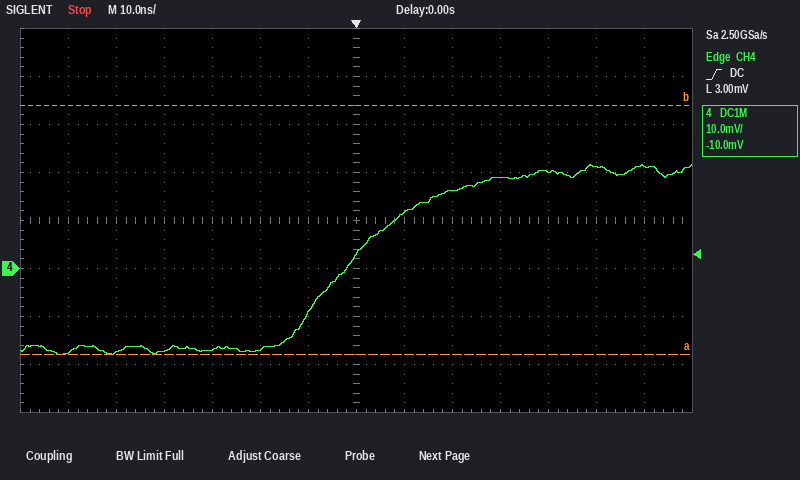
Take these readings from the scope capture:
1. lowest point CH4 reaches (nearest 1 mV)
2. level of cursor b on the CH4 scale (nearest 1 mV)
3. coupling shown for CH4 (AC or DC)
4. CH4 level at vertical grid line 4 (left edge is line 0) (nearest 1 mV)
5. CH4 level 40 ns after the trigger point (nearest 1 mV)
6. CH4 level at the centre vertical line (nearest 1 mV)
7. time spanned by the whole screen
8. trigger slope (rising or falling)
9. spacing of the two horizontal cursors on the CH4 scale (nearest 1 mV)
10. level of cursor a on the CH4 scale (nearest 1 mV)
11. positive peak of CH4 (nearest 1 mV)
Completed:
-18 mV
34 mV
DC
-17 mV
20 mV
3 mV
140 ns
rising
52 mV
-18 mV
22 mV
